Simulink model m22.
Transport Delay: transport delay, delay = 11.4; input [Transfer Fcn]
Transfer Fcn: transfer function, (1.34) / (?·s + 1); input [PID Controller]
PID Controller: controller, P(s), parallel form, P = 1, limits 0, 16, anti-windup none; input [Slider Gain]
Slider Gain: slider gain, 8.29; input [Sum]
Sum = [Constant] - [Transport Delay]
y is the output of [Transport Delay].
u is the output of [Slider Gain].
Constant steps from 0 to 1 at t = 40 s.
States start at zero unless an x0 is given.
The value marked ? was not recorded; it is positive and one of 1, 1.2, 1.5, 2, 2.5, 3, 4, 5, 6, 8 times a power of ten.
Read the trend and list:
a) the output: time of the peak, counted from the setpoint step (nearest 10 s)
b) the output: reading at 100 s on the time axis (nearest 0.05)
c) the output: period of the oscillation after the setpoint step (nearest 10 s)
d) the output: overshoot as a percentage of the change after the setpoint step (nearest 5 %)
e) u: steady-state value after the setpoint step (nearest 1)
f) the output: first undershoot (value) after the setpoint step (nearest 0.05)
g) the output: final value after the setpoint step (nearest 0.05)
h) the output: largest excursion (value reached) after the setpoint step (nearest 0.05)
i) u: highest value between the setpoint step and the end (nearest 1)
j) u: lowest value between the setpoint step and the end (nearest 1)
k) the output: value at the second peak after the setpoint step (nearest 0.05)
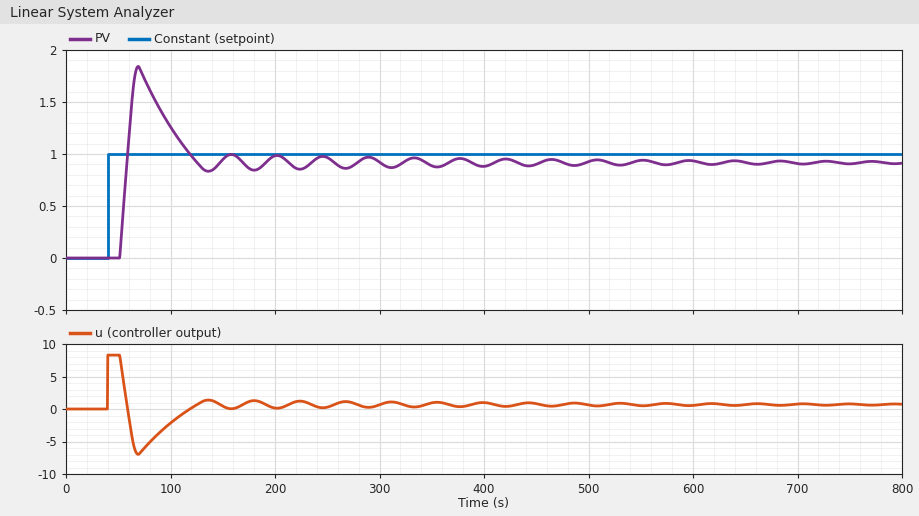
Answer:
30 s
1.25
90 s
100 %
1
0.85
0.90
1.85
8
-7
1.00
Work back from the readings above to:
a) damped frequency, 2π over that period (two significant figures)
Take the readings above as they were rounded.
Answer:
0.070 rad/s
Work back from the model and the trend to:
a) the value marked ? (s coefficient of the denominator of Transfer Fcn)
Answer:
80
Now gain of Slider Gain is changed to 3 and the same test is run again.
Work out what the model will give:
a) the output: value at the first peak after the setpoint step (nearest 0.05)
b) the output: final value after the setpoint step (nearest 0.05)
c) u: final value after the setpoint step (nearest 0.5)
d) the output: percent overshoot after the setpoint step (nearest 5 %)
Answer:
0.90
0.80
0.5
10 %
